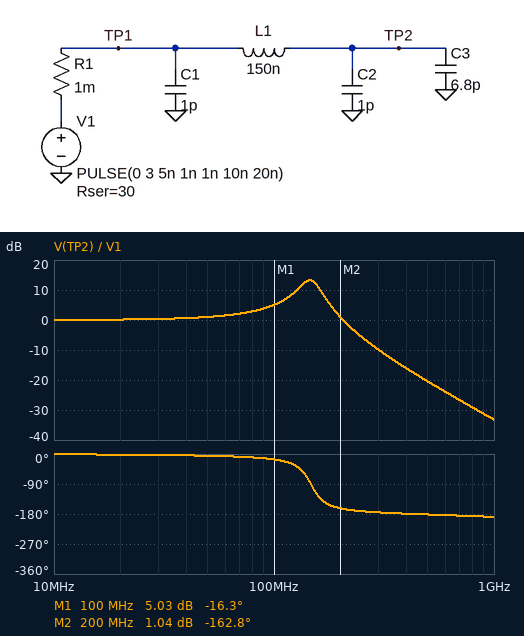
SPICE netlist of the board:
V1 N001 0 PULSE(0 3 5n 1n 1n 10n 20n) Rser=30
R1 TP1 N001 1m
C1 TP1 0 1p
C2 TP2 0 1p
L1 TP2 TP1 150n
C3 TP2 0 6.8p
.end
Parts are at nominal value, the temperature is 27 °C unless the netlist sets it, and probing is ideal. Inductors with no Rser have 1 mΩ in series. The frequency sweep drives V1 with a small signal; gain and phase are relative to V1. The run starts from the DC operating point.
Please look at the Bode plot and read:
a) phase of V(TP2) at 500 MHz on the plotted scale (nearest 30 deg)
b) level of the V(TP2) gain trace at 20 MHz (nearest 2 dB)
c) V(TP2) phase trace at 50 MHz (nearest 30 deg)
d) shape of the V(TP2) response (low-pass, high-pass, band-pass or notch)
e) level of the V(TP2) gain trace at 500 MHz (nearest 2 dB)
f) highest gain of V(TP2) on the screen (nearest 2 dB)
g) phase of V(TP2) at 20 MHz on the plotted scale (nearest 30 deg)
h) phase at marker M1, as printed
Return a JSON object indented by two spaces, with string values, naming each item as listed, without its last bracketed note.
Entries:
{
  "phase of V(TP2) at 500 MHz on the plotted scale": "-180 deg",
  "level of the V(TP2) gain trace at 20 MHz": "0 dB",
  "V(TP2) phase trace at 50 MHz": "0 deg",
  "shape of the V(TP2) response": "low-pass",
  "level of the V(TP2) gain trace at 500 MHz": "-20 dB",
  "highest gain of V(TP2) on the screen": "14 dB",
  "phase of V(TP2) at 20 MHz on the plotted scale": "0 deg",
  "phase at marker M1, as printed": "-16.3 deg"
}
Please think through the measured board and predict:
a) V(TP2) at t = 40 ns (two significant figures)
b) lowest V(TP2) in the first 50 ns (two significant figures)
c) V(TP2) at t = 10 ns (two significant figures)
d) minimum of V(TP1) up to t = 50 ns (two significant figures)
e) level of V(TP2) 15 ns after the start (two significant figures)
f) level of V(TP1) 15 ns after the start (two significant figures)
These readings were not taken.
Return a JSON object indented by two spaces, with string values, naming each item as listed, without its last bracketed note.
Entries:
{
  "V(TP2) at t = 40 ns": "-2.9 V",
  "lowest V(TP2) in the first 50 ns": "-3.0 V",
  "V(TP2) at t = 10 ns": "4.2 V",
  "minimum of V(TP1) up to t = 50 ns": "-550 mV",
  "level of V(TP2) 15 ns after the start": "3.8 V",
  "level of V(TP1) 15 ns after the start": "2.8 V"
}
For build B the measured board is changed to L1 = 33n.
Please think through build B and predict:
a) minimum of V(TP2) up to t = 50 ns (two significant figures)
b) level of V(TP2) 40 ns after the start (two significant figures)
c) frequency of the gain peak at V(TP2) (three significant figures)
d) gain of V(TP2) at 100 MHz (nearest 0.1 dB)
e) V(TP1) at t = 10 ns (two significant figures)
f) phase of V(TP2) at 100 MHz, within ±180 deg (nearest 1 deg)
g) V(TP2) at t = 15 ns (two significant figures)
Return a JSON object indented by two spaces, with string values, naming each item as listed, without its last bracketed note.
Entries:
{
  "minimum of V(TP2) up to t = 50 ns": "-1.2 V",
  "level of V(TP2) 40 ns after the start": "520 mV",
  "frequency of the gain peak at V(TP2)": "300 MHz",
  "gain of V(TP2) at 100 MHz": "0.8 dB",
  "V(TP1) at t = 10 ns": "2.9 V",
  "phase of V(TP2) at 100 MHz, within ±180 deg": "-10 deg",
  "V(TP2) at t = 15 ns": "3.0 V"
}
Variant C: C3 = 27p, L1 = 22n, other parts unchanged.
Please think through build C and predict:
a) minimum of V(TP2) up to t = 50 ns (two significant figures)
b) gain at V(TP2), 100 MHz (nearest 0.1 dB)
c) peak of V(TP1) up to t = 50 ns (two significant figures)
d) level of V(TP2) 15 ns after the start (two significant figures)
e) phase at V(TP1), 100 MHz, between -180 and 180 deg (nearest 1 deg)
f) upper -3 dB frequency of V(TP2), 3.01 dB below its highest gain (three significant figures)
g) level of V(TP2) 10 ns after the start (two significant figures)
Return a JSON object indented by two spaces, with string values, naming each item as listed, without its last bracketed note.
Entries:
{
  "minimum of V(TP2) up to t = 50 ns": "-360 mV",
  "gain at V(TP2), 100 MHz": "0.6 dB",
  "peak of V(TP1) up to t = 50 ns": "3.2 V",
  "level of V(TP2) 15 ns after the start": "3.0 V",
  "phase at V(TP1), 100 MHz, between -180 and 180 deg": "-36 deg",
  "upper -3 dB frequency of V(TP2), 3.01 dB below its highest gain": "238 MHz",
  "level of V(TP2) 10 ns after the start": "3.1 V"
}
